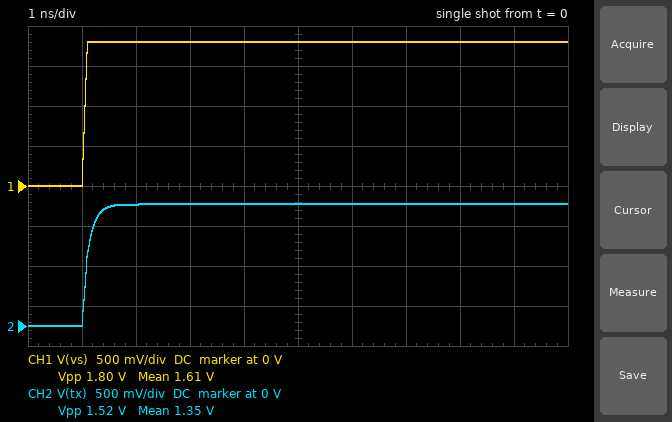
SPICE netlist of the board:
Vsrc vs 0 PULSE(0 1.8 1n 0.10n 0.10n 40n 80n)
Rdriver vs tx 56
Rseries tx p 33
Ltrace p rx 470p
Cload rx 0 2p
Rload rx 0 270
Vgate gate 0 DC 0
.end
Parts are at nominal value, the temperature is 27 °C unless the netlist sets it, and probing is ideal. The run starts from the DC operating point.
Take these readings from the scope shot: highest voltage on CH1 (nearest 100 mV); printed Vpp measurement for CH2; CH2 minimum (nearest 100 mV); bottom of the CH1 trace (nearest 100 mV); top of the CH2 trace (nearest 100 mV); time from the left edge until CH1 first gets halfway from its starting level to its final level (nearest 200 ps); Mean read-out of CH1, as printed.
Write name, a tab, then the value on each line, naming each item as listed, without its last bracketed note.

highest voltage on CH1	1.8 V
printed Vpp measurement for CH2	1.52 V
CH2 minimum	0 V
bottom of the CH1 trace	0 V
top of the CH2 trace	1.5 V
time from the left edge until CH1 first gets halfway from its starting level to its final level	1.0 ns
Mean read-out of CH1, as printed	1.61 V
